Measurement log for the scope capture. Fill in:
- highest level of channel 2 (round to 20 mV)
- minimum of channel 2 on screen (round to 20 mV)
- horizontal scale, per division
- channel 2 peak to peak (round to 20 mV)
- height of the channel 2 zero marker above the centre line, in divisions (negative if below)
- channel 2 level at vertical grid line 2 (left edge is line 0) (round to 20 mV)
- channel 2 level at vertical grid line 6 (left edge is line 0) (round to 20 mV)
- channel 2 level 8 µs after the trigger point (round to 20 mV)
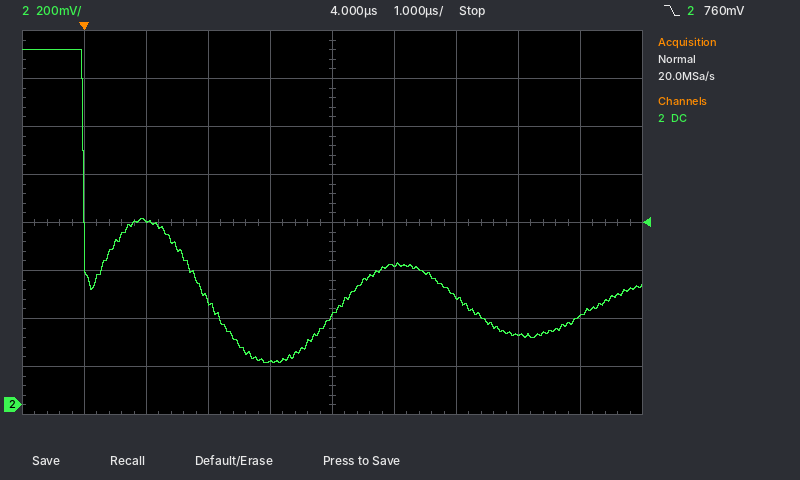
1.48 V
180 mV
1 µs
1.30 V
-3.8 div
760 mV
580 mV
360 mV
